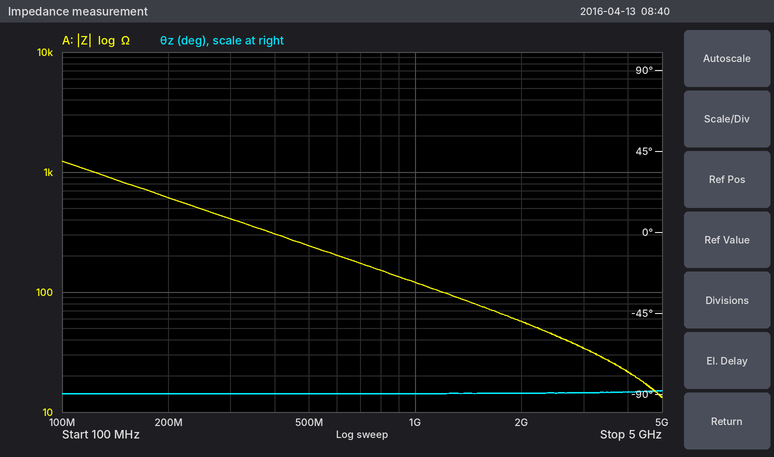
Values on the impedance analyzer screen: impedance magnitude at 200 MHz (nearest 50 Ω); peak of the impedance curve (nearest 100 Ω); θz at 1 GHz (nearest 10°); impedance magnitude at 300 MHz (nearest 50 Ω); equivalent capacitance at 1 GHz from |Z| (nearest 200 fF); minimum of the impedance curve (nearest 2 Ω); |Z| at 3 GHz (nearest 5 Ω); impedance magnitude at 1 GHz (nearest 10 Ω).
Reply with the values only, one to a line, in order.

600 Ω
1.2 kΩ
-90°
400 Ω
1.4 pF
14 Ω
35 Ω
120 Ω
